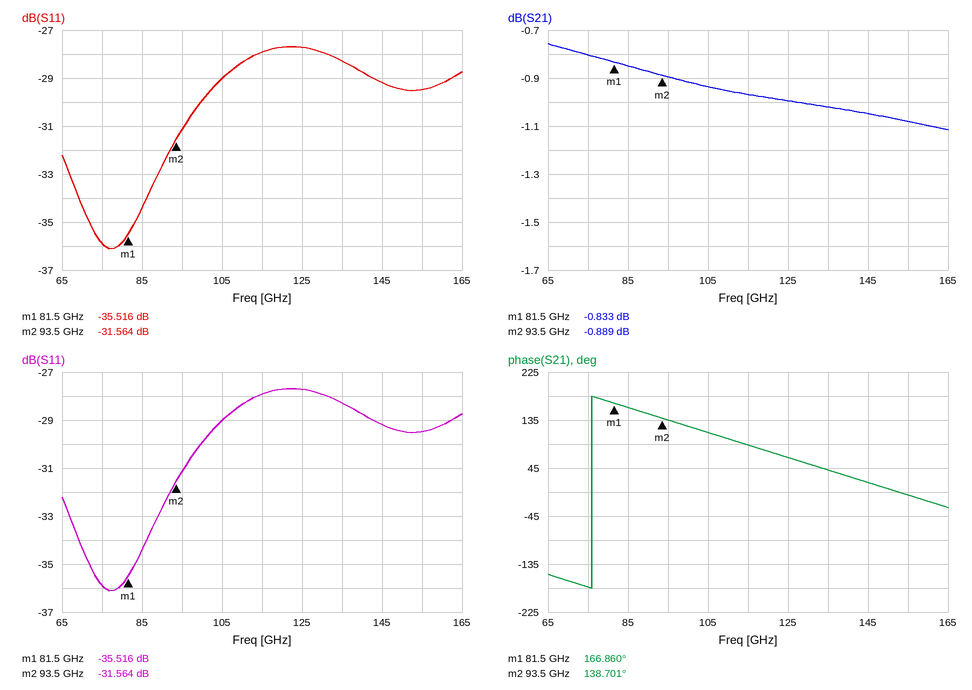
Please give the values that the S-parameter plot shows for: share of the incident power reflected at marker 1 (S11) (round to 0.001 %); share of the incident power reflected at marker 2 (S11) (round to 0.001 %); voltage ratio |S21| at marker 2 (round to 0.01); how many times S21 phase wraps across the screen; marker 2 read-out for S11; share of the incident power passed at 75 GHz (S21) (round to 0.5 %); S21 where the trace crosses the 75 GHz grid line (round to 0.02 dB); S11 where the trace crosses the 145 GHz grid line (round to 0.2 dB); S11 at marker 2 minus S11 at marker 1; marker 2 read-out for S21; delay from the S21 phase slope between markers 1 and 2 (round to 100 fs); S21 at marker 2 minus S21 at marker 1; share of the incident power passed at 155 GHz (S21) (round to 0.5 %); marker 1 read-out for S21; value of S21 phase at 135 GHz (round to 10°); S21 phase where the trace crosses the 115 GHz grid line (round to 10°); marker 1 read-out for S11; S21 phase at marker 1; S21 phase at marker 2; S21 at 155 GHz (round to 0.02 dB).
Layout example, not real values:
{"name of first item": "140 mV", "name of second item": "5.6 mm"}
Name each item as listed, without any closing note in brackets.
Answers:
{"share of the incident power reflected at marker 1 (S11)": "0.028 %", "share of the incident power reflected at marker 2 (S11)": "0.070 %", "voltage ratio |S21| at marker 2": "0.90", "how many times S21 phase wraps across the screen": "1", "marker 2 read-out for S11": "-31.564 dB", "share of the incident power passed at 75 GHz (S21)": "83.0 %", "S21 where the trace crosses the 75 GHz grid line": "-0.80 dB", "S11 where the trace crosses the 145 GHz grid line": "-29.2 dB", "S11 at marker 2 minus S11 at marker 1": "3.952 dB", "marker 2 read-out for S21": "-0.889 dB", "delay from the S21 phase slope between markers 1 and 2": "6.5 ps", "S21 at marker 2 minus S21 at marker 1": "-0.056 dB", "share of the incident power passed at 155 GHz (S21)": "78.0 %", "marker 1 read-out for S21": "-0.833 dB", "value of S21 phase at 135 GHz": "40°", "S21 phase where the trace crosses the 115 GHz grid line": "90°", "marker 1 read-out for S11": "-35.516 dB", "S21 phase at marker 1": "166.860°", "S21 phase at marker 2": "138.701°", "S21 at 155 GHz": "-1.08 dB"}
